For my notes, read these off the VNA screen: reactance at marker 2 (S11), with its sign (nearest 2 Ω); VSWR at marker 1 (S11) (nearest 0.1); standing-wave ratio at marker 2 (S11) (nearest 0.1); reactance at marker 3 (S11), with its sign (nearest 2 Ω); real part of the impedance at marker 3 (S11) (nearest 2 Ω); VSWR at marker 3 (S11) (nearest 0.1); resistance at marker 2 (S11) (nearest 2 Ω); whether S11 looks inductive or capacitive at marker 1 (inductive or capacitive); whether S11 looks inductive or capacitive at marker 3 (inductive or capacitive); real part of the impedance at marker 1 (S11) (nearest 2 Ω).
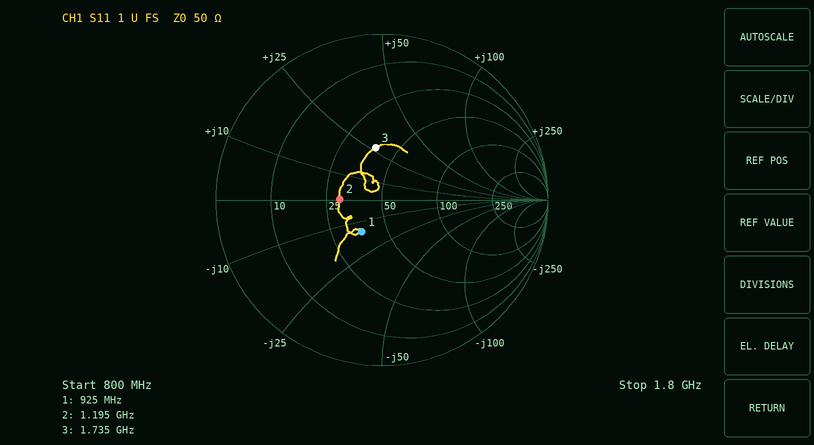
0 Ω
1.6
1.7
+26 Ω
38 Ω
1.9
30 Ω
capacitive
inductive
36 Ω
